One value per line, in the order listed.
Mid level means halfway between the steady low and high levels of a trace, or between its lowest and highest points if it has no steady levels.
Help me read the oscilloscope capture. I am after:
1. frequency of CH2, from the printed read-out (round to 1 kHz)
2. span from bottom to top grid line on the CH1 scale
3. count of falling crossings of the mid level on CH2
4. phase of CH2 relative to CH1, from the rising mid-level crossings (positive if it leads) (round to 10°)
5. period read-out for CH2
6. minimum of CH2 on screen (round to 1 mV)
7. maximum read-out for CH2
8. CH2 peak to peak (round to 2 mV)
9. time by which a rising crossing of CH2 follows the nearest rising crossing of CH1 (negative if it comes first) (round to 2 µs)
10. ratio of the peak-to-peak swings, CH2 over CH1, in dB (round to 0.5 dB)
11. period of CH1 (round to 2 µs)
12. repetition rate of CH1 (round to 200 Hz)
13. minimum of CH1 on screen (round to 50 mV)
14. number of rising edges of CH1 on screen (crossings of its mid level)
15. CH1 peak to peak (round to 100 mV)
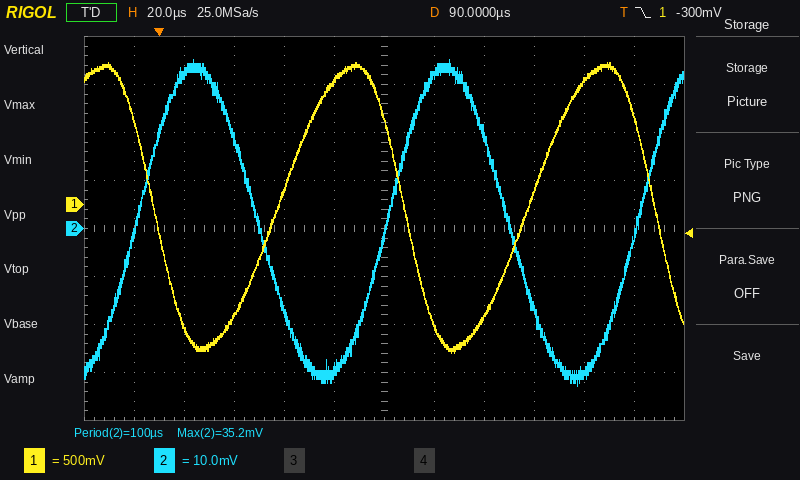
10 kHz
4 V
2
-160°
100 µs
-33 mV
35.2 mV
68 mV
+44 µs
-33.0 dB
100 µs
10.0 kHz
-1.55 V
2
3.00 V
